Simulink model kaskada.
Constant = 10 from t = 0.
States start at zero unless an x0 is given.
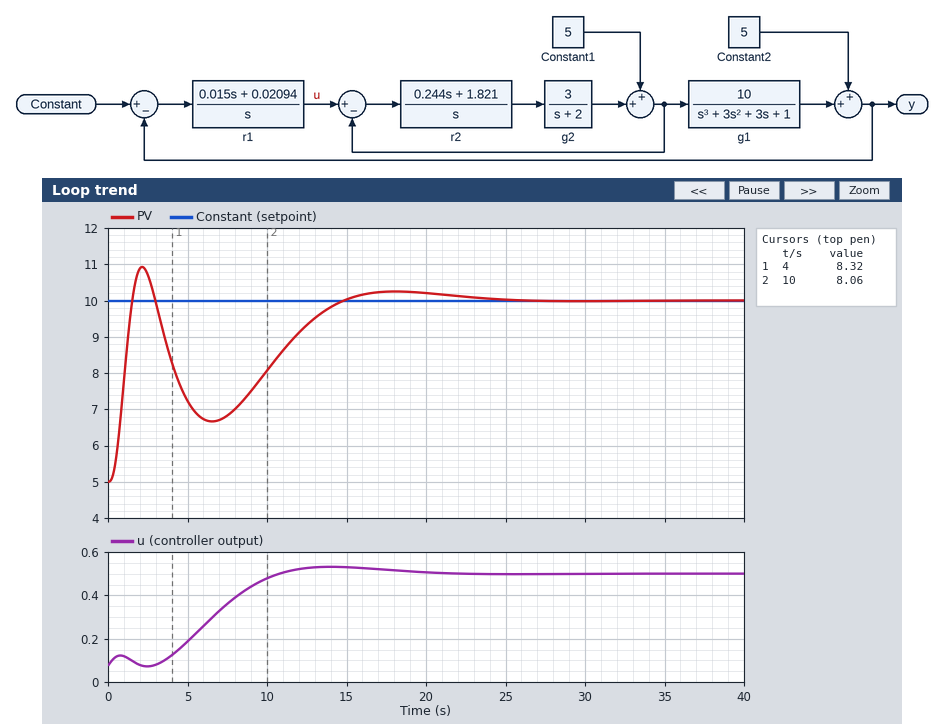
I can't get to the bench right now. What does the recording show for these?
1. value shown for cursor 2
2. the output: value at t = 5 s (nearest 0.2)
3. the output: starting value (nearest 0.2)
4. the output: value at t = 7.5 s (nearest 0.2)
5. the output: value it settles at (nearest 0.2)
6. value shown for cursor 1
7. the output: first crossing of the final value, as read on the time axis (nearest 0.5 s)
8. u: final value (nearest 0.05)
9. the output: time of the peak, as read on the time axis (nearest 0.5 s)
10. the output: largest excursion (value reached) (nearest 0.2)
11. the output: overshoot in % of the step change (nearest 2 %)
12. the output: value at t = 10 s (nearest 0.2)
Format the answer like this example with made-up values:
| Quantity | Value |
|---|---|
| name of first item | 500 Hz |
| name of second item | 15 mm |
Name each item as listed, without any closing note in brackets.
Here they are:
| Quantity | Value |
|---|---|
| value shown for cursor 2 | 8.06 |
| the output: value at t = 5 s | 7.2 |
| the output: starting value | 5.0 |
| the output: value at t = 7.5 s | 6.8 |
| the output: value it settles at | 10.0 |
| value shown for cursor 1 | 8.32 |
| the output: first crossing of the final value, as read on the time axis | 1.5 s |
| u: final value | 0.50 |
| the output: time of the peak, as read on the time axis | 2.0 s |
| the output: largest excursion (value reached) | 11.0 |
| the output: overshoot in % of the step change | 18 % |
| the output: value at t = 10 s | 8.0 |
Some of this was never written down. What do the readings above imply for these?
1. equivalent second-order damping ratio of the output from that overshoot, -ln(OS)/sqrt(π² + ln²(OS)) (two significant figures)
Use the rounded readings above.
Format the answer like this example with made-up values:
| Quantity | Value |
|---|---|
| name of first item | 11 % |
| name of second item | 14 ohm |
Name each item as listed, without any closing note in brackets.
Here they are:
| Quantity | Value |
|---|---|
| equivalent second-order damping ratio of the output from that overshoot, -ln(OS)/sqrt(π² + ln²(OS)) | 0.48 |
